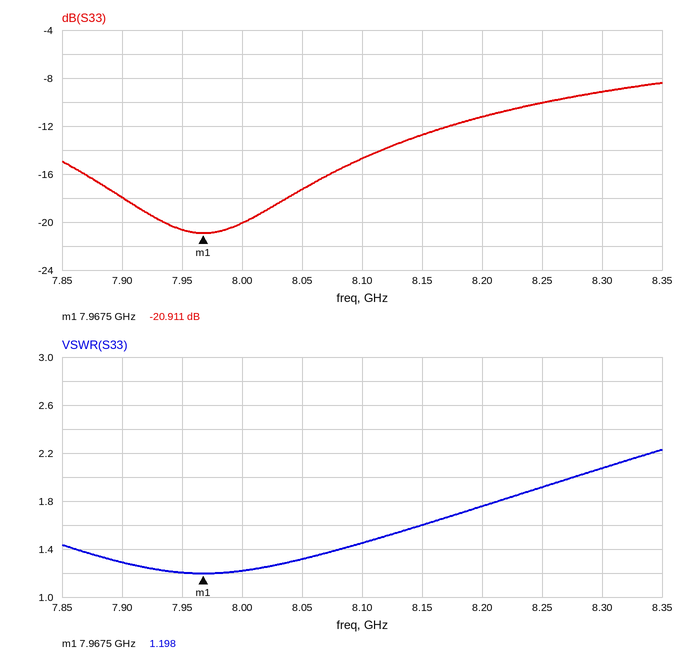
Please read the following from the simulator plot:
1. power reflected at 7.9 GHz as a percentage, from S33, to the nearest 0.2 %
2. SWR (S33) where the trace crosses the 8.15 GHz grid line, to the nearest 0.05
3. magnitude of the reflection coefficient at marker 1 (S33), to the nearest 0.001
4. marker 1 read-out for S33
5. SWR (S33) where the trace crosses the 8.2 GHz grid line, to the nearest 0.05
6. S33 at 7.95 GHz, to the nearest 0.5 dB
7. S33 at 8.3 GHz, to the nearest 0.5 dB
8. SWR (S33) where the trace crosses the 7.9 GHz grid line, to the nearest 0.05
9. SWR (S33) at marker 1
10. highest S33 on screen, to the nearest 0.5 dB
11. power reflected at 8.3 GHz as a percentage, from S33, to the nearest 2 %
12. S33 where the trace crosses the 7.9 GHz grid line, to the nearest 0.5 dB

1.6 %
1.60
0.090
-20.911 dB
1.75
-20.5 dB
-9.0 dB
1.30
1.198
-8.5 dB
12 %
-18.0 dB
